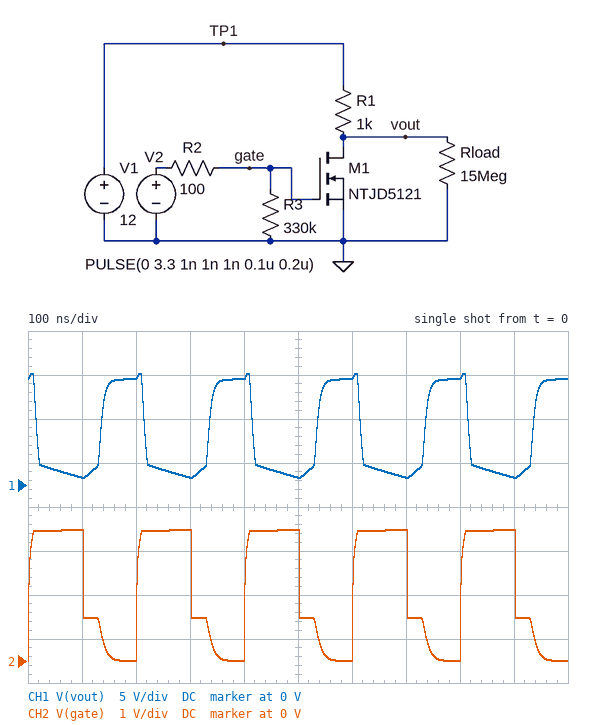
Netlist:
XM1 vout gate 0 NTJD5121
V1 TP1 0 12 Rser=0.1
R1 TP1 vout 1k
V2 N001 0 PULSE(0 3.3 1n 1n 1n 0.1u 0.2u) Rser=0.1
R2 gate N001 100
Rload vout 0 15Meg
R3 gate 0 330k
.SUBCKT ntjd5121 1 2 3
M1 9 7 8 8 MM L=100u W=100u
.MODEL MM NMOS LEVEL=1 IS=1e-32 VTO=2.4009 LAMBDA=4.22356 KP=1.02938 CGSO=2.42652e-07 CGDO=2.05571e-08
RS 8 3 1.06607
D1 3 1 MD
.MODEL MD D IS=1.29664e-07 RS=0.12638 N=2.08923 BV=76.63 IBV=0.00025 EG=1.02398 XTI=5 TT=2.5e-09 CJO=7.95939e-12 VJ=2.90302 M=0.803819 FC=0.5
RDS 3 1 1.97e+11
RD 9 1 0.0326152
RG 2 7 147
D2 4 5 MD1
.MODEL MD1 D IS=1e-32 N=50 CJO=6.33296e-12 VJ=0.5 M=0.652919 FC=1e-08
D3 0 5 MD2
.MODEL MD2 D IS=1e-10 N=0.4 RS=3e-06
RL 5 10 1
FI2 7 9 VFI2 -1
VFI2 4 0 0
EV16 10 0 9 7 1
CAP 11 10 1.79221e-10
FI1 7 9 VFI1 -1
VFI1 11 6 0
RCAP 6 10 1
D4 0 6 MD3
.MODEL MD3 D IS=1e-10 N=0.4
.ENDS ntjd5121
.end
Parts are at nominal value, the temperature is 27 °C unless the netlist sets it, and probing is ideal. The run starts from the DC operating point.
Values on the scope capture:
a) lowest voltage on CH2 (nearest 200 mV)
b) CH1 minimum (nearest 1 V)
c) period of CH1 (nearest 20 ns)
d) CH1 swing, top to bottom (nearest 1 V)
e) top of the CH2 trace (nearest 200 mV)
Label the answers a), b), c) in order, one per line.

a) 0 V
b) 1 V
c) 200 ns
d) 12 V
e) 3.0 V
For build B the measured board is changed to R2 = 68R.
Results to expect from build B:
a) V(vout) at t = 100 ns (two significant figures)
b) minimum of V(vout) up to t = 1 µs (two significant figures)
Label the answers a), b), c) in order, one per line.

a) 590 mV
b) 490 mV
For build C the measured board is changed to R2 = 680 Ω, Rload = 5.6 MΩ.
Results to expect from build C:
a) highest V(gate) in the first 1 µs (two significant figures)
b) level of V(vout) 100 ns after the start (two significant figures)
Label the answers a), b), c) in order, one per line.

a) 2.6 V
b) 2.1 V
